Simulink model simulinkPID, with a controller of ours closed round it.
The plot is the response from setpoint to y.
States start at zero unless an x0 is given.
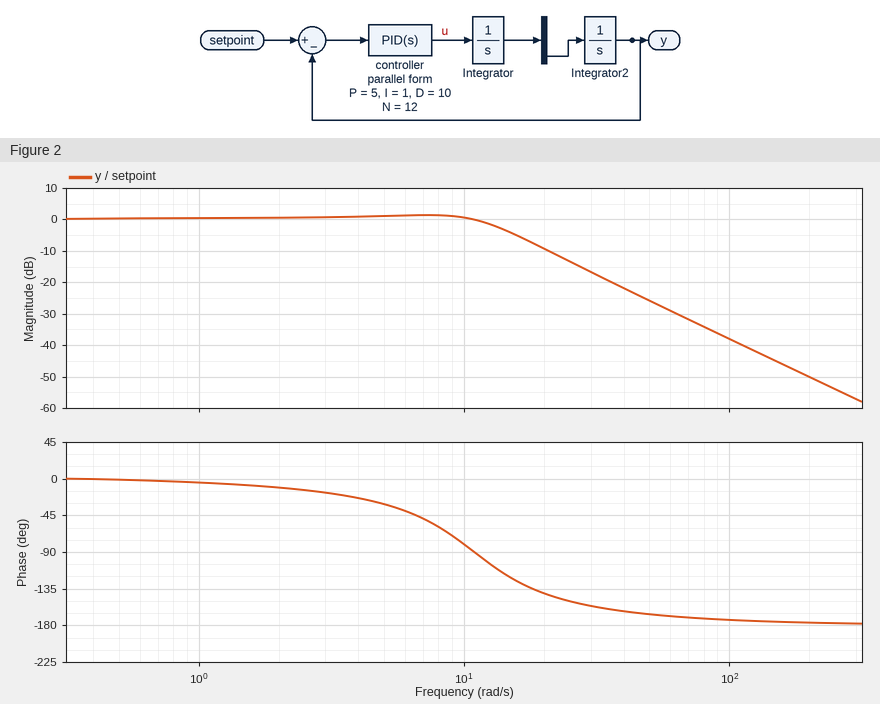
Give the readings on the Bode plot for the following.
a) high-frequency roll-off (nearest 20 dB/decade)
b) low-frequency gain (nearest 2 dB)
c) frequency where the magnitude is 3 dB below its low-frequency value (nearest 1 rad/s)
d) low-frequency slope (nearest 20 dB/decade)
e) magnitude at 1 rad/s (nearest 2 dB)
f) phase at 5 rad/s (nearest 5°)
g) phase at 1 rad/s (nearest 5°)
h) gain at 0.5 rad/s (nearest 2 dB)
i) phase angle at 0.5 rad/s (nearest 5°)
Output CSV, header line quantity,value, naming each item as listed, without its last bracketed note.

quantity,value
high-frequency roll-off,-40 dB/decade
low-frequency gain,0 dB
frequency where the magnitude is 3 dB below its low-frequency value,14 rad/s
low-frequency slope,0 dB/decade
magnitude at 1 rad/s,0 dB
phase at 5 rad/s,-30°
phase at 1 rad/s,-5°
gain at 0.5 rad/s,0 dB
phase angle at 0.5 rad/s,0°
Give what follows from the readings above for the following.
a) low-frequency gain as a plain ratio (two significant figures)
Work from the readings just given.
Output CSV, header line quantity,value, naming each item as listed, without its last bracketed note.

quantity,value
low-frequency gain as a plain ratio,1.0
